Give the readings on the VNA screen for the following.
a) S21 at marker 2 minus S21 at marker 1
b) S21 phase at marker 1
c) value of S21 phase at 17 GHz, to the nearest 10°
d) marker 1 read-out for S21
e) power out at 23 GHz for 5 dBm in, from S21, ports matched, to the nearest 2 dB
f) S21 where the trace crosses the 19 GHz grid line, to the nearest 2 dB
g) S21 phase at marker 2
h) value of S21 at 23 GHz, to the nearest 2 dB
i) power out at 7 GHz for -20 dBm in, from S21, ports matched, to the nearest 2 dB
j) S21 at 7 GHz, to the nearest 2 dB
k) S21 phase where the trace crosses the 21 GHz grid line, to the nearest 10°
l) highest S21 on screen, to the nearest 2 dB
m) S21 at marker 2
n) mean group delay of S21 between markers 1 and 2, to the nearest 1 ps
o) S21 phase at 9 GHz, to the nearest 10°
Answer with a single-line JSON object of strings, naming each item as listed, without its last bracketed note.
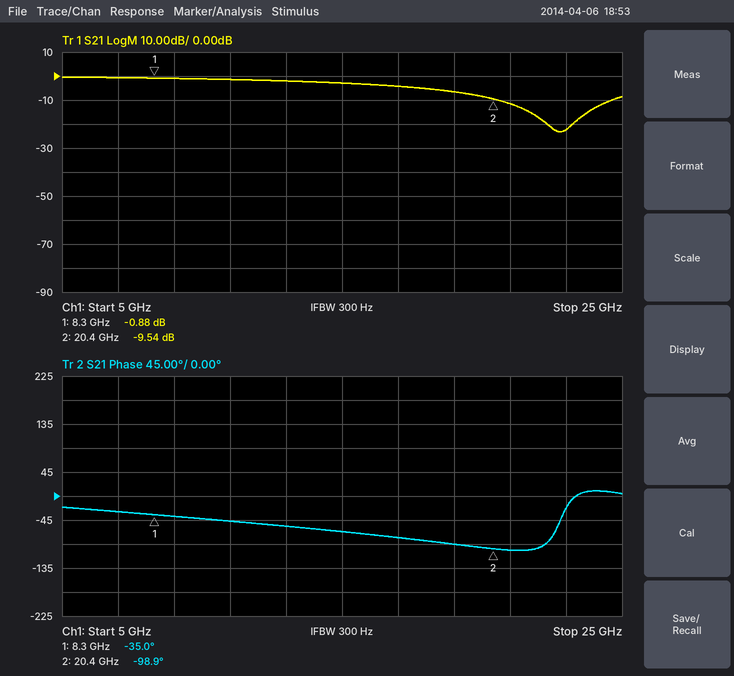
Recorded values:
{"S21 at marker 2 minus S21 at marker 1": "-8.66 dB", "S21 phase at marker 1": "-35.0°", "value of S21 phase at 17 GHz, to the nearest 10°": "-80°", "marker 1 read-out for S21": "-0.88 dB", "power out at 23 GHz for 5 dBm in, from S21, ports matched, to the nearest 2 dB": "-18 dBm", "S21 where the trace crosses the 19 GHz grid line, to the nearest 2 dB": "-6 dB", "S21 phase at marker 2": "-98.9°", "value of S21 at 23 GHz, to the nearest 2 dB": "-22 dB", "power out at 7 GHz for -20 dBm in, from S21, ports matched, to the nearest 2 dB": "-20 dBm", "S21 at 7 GHz, to the nearest 2 dB": "0 dB", "S21 phase where the trace crosses the 21 GHz grid line, to the nearest 10°": "-100°", "highest S21 on screen, to the nearest 2 dB": "0 dB", "S21 at marker 2": "-9.54 dB", "mean group delay of S21 between markers 1 and 2, to the nearest 1 ps": "15 ps", "S21 phase at 9 GHz, to the nearest 10°": "-40°"}
